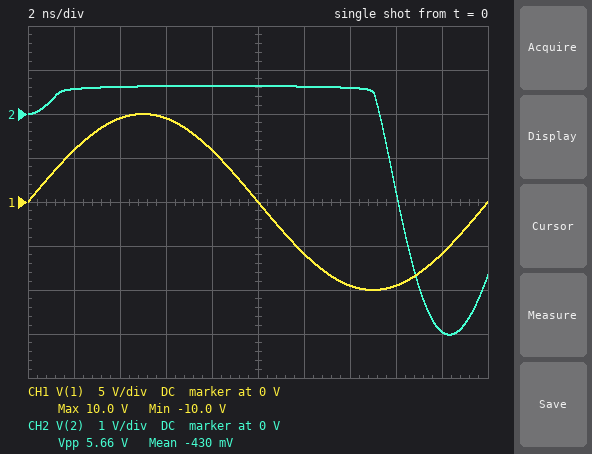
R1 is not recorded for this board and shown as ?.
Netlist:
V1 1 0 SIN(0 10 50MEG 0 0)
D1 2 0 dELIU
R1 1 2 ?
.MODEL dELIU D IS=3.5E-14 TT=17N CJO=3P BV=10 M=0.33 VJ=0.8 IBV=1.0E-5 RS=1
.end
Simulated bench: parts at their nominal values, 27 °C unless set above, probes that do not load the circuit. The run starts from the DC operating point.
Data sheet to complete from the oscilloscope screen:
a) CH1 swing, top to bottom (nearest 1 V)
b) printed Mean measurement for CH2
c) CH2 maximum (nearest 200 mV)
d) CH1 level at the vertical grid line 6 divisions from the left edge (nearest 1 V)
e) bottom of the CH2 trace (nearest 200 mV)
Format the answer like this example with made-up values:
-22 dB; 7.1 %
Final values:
20 V; -430 mV; 600 mV; -6 V; -5.0 V
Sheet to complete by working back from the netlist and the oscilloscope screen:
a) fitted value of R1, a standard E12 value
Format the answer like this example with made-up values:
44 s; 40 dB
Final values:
1.5 kΩ
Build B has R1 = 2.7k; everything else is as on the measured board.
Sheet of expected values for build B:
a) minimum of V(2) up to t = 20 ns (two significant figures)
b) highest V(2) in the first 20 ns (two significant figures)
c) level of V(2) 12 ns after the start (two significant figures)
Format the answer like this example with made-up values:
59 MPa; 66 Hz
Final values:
-3.2 V; 620 mV; 610 mV
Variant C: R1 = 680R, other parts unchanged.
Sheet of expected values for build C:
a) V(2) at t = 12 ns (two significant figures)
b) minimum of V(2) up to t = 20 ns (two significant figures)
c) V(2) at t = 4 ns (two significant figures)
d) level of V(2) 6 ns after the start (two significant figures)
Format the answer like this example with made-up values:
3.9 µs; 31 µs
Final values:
640 mV; -7.4 V; 650 mV; 660 mV
